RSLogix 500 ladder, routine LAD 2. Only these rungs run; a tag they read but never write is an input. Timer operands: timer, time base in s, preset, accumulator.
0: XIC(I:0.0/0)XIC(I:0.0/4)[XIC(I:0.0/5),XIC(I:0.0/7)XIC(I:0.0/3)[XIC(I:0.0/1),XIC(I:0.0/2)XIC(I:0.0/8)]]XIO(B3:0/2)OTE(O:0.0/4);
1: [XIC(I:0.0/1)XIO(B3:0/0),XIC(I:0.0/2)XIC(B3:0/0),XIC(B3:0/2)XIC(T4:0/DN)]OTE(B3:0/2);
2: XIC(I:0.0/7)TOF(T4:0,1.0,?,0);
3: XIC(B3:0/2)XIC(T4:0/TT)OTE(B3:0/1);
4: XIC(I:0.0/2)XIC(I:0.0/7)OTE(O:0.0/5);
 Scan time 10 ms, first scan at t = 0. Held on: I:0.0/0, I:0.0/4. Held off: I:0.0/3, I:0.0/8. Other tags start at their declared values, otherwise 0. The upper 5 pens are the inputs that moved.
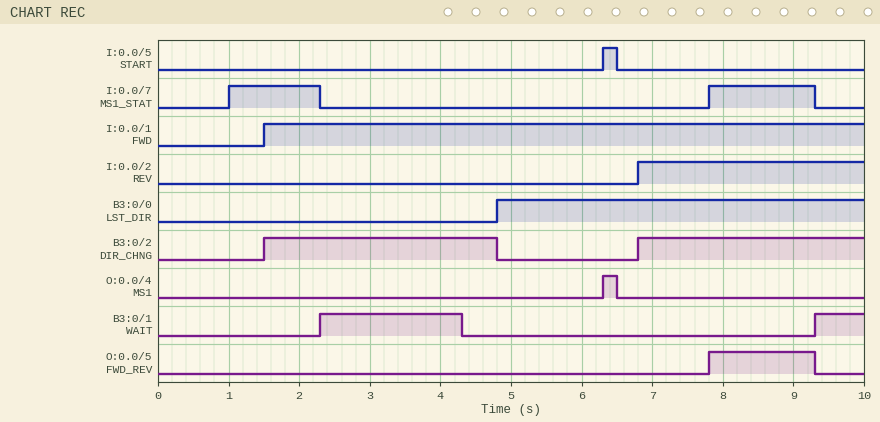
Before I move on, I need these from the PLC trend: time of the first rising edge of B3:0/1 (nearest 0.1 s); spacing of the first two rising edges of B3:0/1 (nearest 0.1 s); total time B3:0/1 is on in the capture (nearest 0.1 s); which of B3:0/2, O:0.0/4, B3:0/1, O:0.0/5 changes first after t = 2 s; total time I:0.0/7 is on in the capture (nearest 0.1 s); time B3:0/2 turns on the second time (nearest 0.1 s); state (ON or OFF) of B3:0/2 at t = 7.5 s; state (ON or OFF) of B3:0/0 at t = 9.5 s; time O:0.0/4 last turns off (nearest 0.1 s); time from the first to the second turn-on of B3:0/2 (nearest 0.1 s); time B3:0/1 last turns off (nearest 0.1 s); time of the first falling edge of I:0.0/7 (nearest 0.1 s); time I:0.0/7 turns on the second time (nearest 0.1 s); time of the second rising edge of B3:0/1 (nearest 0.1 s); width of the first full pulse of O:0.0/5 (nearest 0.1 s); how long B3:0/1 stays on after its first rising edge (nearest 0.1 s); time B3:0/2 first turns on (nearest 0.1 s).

2.3 s
7.0 s
2.7 s
B3:0/1
2.8 s
6.8 s
ON
ON
6.5 s
5.3 s
4.3 s
2.3 s
7.8 s
9.3 s
1.5 s
2.0 s
1.5 s
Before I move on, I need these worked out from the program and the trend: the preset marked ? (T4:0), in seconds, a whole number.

2 s
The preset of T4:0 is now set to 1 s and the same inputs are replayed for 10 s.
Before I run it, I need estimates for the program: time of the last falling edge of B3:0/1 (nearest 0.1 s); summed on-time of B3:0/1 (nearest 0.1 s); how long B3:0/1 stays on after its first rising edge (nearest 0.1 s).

3.3 s
1.7 s
1.0 s
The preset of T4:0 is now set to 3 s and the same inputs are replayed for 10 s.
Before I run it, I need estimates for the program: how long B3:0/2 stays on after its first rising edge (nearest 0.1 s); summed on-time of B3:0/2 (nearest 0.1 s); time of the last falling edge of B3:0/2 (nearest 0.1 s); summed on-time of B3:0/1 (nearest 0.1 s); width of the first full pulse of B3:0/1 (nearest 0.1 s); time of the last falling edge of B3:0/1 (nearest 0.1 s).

3.8 s
7.0 s
5.3 s
3.7 s
3.0 s
5.3 s
